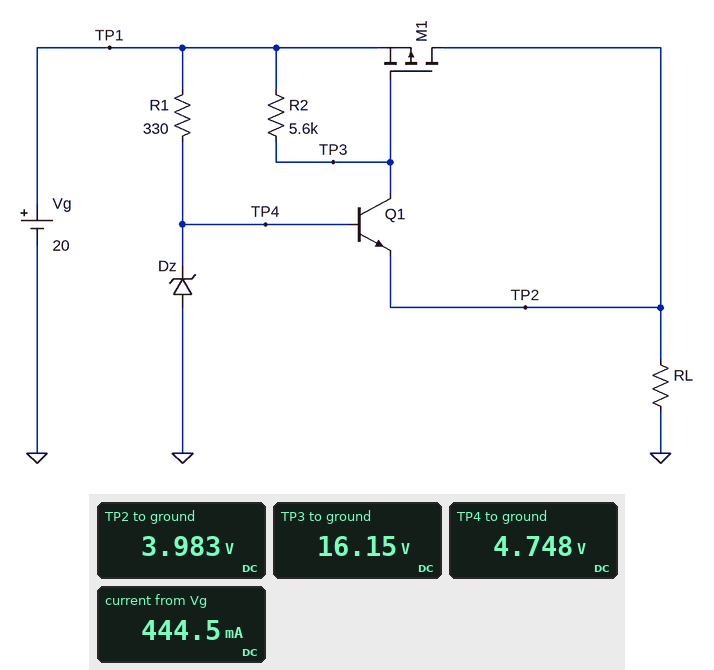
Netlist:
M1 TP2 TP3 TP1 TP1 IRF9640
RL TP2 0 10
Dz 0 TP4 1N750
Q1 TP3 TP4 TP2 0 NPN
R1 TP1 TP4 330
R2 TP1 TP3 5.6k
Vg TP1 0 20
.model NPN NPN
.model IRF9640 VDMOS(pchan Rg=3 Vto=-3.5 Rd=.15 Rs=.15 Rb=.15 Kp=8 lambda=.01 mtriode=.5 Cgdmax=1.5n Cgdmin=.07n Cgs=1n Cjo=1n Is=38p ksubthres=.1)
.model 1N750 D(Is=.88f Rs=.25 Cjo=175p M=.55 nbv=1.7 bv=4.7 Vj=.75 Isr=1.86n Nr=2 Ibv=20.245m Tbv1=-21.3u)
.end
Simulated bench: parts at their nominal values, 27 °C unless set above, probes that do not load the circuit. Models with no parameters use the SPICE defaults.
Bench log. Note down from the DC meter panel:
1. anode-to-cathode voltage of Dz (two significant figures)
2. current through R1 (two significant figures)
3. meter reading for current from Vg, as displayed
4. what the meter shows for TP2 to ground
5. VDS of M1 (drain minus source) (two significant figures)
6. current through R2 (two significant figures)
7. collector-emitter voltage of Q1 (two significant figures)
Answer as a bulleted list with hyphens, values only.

- -4.7 V
- 46 mA
- 444.5 mA
- 3.983 V
- -16 V
- 690 µA
- 12 V
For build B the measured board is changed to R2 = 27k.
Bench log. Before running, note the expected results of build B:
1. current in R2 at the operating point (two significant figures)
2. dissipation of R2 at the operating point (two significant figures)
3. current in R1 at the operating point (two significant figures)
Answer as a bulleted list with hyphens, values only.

- 140 µA
- 550 µW
- 46 mA
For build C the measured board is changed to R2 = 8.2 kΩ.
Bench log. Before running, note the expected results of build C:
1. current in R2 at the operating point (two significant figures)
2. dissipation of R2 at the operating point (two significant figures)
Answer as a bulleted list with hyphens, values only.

- 470 µA
- 1.8 mW
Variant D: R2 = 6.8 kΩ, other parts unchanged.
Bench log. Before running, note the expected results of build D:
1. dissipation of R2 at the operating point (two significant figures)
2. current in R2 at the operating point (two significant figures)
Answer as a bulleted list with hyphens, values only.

- 2.2 mW
- 570 µA
